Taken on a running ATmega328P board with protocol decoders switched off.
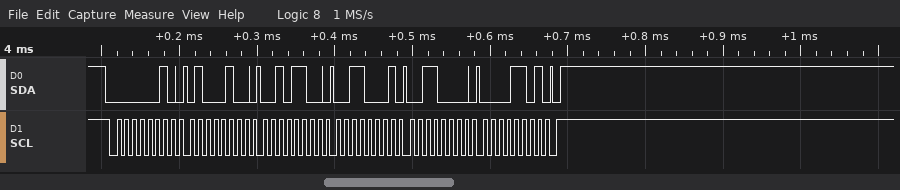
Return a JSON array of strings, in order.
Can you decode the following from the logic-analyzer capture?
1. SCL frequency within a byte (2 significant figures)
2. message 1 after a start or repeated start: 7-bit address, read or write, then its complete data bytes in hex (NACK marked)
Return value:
["100 kHz", "0x01 write: 44 2C 31 30 0D"]
